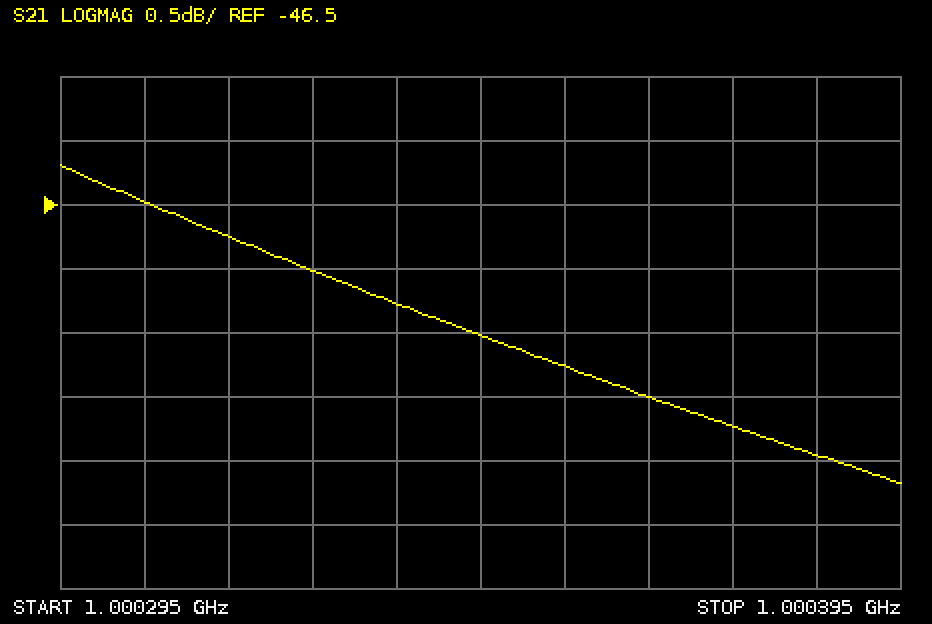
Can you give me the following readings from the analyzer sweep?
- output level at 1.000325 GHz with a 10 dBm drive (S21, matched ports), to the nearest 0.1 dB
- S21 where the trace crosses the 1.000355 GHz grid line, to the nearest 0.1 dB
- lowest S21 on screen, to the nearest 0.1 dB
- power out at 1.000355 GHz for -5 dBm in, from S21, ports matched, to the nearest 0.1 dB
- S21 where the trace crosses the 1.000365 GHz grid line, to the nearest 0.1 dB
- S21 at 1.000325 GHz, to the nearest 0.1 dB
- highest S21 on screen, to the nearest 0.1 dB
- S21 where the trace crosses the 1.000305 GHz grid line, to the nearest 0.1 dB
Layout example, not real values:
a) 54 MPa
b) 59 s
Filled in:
a) -37.0 dBm
b) -47.8 dB
c) -48.7 dB
d) -52.8 dBm
e) -48.0 dB
f) -47.0 dB
g) -46.2 dB
h) -46.5 dB
